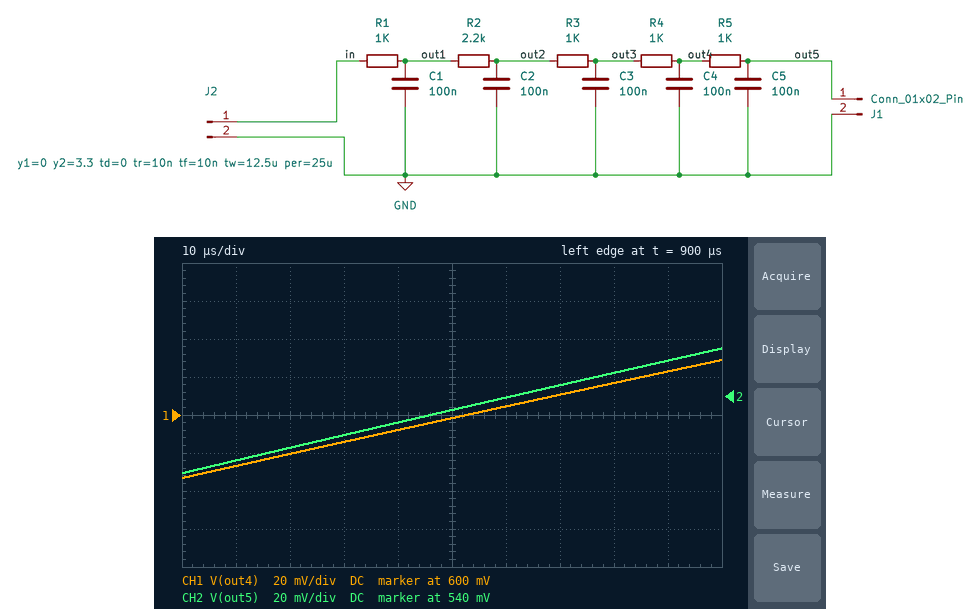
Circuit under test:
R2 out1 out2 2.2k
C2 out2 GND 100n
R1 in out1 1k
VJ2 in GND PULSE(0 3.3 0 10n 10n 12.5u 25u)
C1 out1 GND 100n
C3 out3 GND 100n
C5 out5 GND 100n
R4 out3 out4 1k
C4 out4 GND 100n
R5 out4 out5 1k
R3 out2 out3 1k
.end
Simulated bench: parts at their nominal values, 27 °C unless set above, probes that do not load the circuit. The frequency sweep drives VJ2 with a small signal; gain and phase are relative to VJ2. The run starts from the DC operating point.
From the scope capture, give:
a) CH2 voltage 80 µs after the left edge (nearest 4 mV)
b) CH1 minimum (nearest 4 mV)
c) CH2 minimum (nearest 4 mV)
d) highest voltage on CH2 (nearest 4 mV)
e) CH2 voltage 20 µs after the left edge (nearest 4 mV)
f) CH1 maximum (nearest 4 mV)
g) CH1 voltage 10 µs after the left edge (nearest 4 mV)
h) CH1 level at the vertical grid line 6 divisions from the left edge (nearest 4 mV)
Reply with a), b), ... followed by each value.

a) 552 mV
b) 568 mV
c) 500 mV
d) 564 mV
e) 512 mV
f) 628 mV
g) 572 mV
h) 604 mV
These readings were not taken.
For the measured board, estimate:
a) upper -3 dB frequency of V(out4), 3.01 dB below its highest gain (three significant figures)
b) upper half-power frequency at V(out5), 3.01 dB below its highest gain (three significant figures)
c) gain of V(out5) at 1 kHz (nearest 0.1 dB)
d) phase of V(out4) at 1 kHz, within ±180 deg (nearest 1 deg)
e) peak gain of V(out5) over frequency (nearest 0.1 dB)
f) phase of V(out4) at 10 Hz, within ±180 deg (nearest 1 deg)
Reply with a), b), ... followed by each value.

a) 93.6 Hz
b) 93.2 Hz
c) -24.5 dB
d) -145 deg
e) 0 dB
f) -7 deg
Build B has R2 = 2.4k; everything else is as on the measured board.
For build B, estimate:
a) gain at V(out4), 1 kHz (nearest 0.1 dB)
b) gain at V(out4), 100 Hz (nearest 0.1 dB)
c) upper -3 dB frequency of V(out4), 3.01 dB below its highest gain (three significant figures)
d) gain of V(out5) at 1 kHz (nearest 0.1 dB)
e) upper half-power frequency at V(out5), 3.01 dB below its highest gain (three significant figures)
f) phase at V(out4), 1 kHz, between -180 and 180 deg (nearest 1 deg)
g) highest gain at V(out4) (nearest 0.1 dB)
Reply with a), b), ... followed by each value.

a) -23.5 dB
b) -3.5 dB
c) 89.5 Hz
d) -24.9 dB
e) 89.2 Hz
f) -146 deg
g) 0 dB
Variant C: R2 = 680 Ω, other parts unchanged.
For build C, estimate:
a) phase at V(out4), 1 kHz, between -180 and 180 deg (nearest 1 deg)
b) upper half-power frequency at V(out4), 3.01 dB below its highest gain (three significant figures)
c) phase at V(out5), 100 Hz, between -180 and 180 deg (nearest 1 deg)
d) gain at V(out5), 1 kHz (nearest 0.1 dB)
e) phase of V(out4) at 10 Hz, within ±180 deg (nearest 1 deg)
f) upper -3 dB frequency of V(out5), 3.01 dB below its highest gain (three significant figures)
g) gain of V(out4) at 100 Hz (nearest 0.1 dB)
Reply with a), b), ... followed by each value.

a) -131 deg
b) 141 Hz
c) -44 deg
d) -20.4 dB
e) -5 deg
f) 140 Hz
g) -1.8 dB
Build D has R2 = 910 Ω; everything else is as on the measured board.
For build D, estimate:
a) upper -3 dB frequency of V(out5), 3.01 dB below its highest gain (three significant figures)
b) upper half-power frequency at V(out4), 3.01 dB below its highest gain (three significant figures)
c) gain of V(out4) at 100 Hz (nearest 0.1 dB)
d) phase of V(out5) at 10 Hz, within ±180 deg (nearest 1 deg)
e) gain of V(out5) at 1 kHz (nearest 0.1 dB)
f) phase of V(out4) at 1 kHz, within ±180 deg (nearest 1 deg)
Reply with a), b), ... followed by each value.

a) 130 Hz
b) 131 Hz
c) -2.0 dB
d) -5 deg
e) -21.1 dB
f) -134 deg
